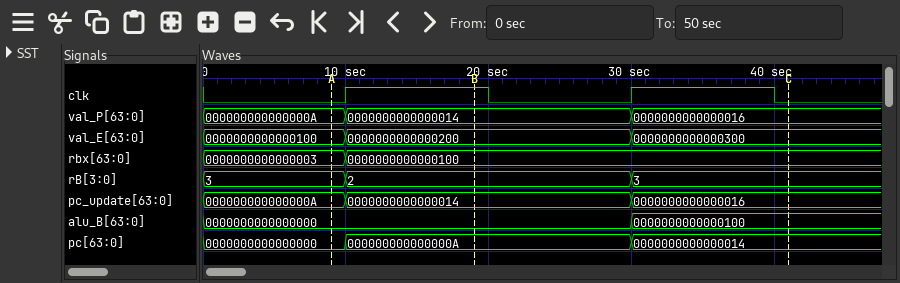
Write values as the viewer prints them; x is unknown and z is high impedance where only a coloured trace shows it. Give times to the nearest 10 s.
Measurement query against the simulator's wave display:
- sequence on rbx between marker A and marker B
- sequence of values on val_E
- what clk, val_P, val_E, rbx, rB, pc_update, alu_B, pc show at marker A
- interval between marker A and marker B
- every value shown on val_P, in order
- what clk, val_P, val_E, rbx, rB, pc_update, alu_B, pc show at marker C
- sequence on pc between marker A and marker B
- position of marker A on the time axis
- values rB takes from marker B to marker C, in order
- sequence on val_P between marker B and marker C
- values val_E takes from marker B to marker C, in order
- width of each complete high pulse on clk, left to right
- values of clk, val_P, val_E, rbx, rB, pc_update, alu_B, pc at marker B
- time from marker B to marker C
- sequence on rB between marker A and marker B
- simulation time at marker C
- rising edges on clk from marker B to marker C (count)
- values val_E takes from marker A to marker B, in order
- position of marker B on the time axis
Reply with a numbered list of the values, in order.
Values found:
1. 0000000000000003, 0000000000000100
2. 0000000000000100, 0000000000000200, 0000000000000300
3. clk=0, val_P=000000000000000A, val_E=0000000000000100, rbx=0000000000000003, rB=3, pc_update=000000000000000A, alu_B=0000000000000000, pc=0000000000000000
4. 10 s
5. 000000000000000A, 0000000000000014, 0000000000000016
6. clk=0, val_P=0000000000000016, val_E=0000000000000300, rbx=0000000000000100, rB=3, pc_update=0000000000000016, alu_B=0000000000000100, pc=0000000000000014
7. 0000000000000000, 000000000000000A
8. 10 s
9. 2, 3
10. 0000000000000014, 0000000000000016
11. 0000000000000200, 0000000000000300
12. 10 s, 10 s
13. clk=1, val_P=0000000000000014, val_E=0000000000000200, rbx=0000000000000100, rB=2, pc_update=0000000000000014, alu_B=0000000000000000, pc=000000000000000A
14. 20 s
15. 3, 2
16. 40 s
17. 1
18. 0000000000000100, 0000000000000200
19. 20 s
